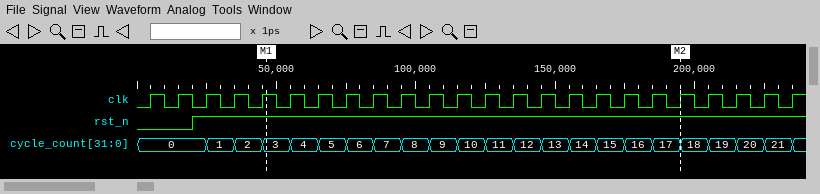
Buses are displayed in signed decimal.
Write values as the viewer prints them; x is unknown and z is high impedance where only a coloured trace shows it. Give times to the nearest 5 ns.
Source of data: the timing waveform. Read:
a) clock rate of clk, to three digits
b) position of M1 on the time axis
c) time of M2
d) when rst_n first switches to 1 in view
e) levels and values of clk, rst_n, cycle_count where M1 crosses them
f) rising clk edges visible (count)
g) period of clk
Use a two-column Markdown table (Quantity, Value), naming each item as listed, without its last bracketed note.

| Quantity | Value |
|---|---|
| clock rate of clk, to three digits | 100 MHz |
| position of M1 on the time axis | 45 ns |
| time of M2 | 195 ns |
| when rst_n first switches to 1 in view | 20 ns |
| levels and values of clk, rst_n, cycle_count where M1 crosses them | clk=1, rst_n=1, cycle_count=3 |
| rising clk edges visible | 24 |
| period of clk | 10 ns |
